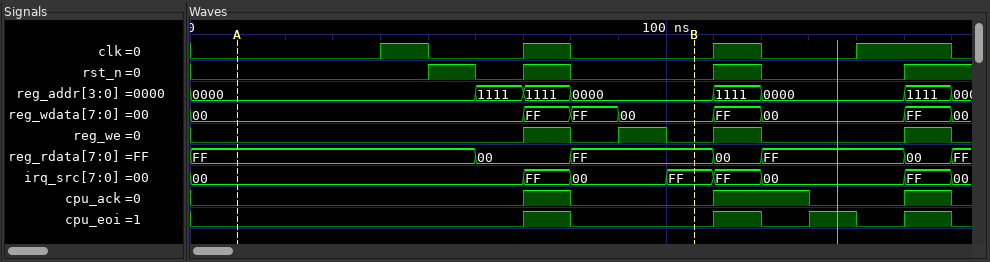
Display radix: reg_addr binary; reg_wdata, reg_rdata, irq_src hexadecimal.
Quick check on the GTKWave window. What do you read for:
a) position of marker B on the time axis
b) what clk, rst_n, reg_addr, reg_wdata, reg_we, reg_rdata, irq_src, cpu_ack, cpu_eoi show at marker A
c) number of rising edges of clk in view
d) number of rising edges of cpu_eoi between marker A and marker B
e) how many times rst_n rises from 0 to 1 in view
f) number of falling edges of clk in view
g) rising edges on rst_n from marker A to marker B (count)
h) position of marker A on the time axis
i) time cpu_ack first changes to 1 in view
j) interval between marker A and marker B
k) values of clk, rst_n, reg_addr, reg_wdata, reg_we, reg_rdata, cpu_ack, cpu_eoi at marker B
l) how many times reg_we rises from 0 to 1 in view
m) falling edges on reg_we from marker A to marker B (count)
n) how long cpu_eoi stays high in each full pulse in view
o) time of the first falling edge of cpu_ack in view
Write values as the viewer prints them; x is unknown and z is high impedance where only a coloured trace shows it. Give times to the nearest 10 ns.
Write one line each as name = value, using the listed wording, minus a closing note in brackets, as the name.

position of marker B on the time axis = 110 ns
what clk, rst_n, reg_addr, reg_wdata, reg_we, reg_rdata, irq_src, cpu_ack, cpu_eoi show at marker A = clk=0, rst_n=0, reg_addr=0000, reg_wdata=00, reg_we=0, reg_rdata=FF, irq_src=00, cpu_ack=0, cpu_eoi=0
number of rising edges of clk in view = 4
number of rising edges of cpu_eoi between marker A and marker B = 1
how many times rst_n rises from 0 to 1 in view = 4
number of falling edges of clk in view = 4
rising edges on rst_n from marker A to marker B = 2
position of marker A on the time axis = 10 ns
time cpu_ack first changes to 1 in view = 70 ns
interval between marker A and marker B = 100 ns
values of clk, rst_n, reg_addr, reg_wdata, reg_we, reg_rdata, cpu_ack, cpu_eoi at marker B = clk=0, rst_n=0, reg_addr=0000, reg_wdata=00, reg_we=0, reg_rdata=FF, cpu_ack=0, cpu_eoi=0
how many times reg_we rises from 0 to 1 in view = 4
falling edges on reg_we from marker A to marker B = 2
how long cpu_eoi stays high in each full pulse in view = 10 ns, 10 ns, 10 ns, 10 ns
time of the first falling edge of cpu_ack in view = 80 ns
